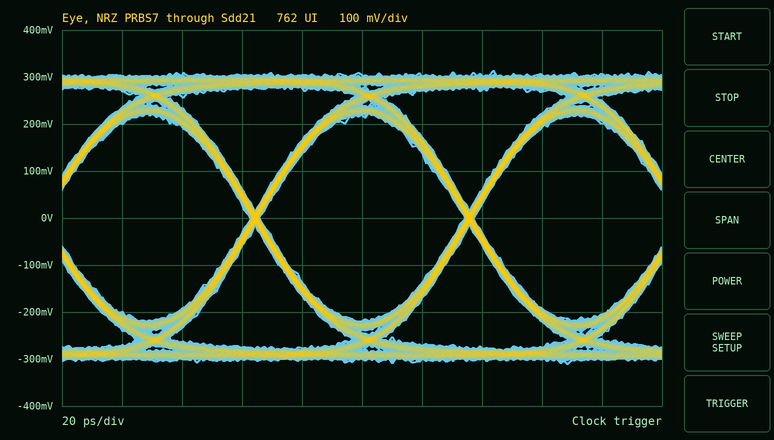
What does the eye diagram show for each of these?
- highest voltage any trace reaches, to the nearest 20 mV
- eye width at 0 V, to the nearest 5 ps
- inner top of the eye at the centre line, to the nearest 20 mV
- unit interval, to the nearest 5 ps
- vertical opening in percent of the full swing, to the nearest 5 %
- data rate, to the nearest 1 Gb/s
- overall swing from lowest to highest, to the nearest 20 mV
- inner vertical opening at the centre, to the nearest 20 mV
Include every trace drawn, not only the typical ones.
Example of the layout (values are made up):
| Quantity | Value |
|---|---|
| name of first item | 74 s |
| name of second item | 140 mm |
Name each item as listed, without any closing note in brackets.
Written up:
| Quantity | Value |
|---|---|
| highest voltage any trace reaches, to the nearest 20 mV | 320 mV |
| eye width at 0 V, to the nearest 5 ps | 70 ps |
| inner top of the eye at the centre line, to the nearest 20 mV | 220 mV |
| unit interval, to the nearest 5 ps | 70 ps |
| vertical opening in percent of the full swing, to the nearest 5 % | 70 % |
| data rate, to the nearest 1 Gb/s | 14 Gb/s |
| overall swing from lowest to highest, to the nearest 20 mV | 620 mV |
| inner vertical opening at the centre, to the nearest 20 mV | 440 mV |
